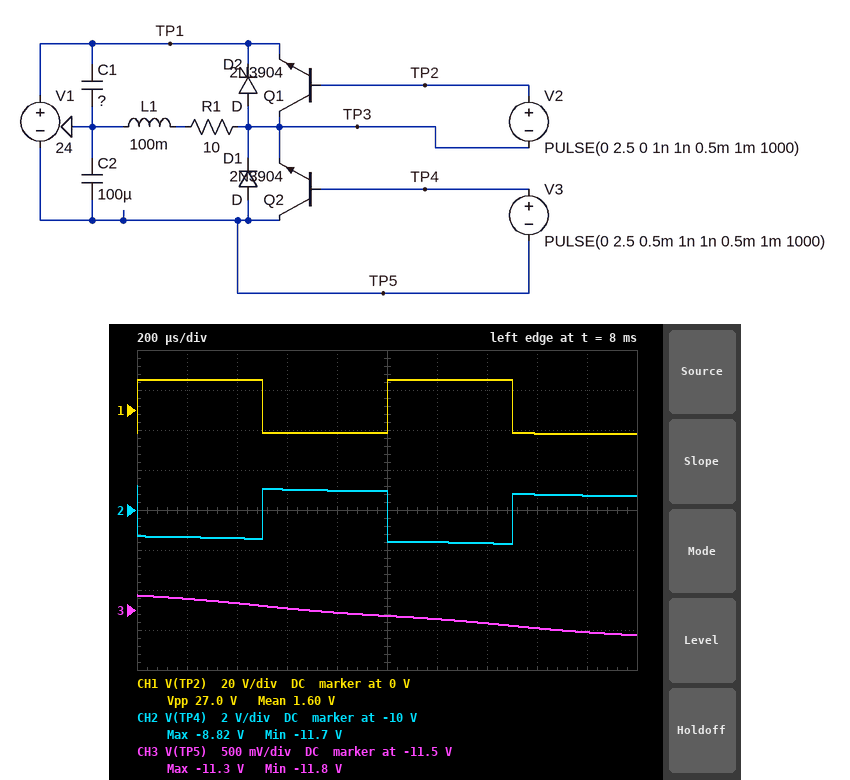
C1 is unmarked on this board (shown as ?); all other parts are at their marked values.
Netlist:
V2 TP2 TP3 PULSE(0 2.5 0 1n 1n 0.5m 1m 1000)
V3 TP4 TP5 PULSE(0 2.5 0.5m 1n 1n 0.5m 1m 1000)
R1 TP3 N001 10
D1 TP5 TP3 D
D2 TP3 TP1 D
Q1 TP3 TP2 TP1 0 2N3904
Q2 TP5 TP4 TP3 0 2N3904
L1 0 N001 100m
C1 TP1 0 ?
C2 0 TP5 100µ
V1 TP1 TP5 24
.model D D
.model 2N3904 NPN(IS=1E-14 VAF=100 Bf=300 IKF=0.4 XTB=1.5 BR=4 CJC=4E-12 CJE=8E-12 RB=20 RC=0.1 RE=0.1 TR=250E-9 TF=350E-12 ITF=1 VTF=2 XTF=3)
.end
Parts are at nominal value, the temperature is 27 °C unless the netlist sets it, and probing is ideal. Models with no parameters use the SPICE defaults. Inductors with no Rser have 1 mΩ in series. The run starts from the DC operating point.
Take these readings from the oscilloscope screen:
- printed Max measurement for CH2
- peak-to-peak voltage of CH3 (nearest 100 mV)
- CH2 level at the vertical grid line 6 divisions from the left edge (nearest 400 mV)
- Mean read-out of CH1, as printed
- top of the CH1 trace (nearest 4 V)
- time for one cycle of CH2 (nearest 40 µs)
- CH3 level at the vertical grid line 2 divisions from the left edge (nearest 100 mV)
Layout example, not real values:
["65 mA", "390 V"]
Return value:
["-8.82 V", "500 mV", "-11.6 V", "1.60 V", "16 V", "1.00 ms", "-11.4 V"]
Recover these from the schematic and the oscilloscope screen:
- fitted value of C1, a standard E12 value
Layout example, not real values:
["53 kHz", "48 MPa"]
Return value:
["270 µF"]
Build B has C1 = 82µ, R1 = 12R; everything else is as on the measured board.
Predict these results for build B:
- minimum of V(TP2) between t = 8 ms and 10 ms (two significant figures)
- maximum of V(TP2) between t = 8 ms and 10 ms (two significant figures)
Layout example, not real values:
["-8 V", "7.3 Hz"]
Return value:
["-13 V", "14 V"]
